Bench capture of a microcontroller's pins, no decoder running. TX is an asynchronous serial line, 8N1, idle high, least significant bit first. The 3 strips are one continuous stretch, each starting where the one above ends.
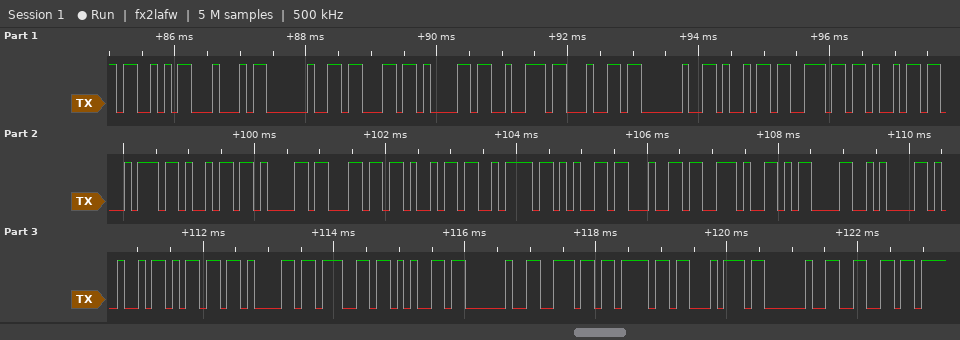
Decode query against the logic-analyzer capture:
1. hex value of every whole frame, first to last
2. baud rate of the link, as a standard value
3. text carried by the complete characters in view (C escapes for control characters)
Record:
53 44 20 63 61 72 64 20 69 6E 69 74 69 61 6C 69 7A 65 64 2E 0D 0A 49 6D 61 67 65 20 6E 6F 74 20 66
9600 baud
"SD card initialized.\r\nImage not f"
